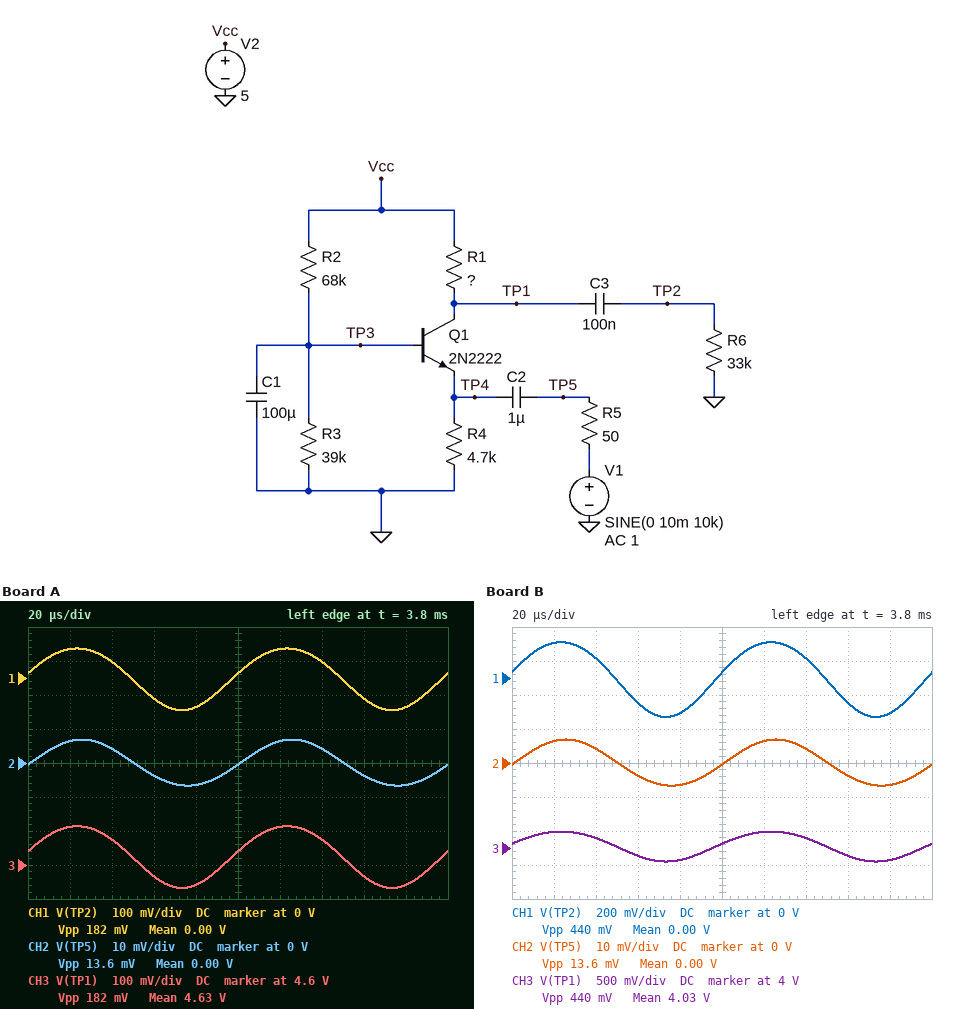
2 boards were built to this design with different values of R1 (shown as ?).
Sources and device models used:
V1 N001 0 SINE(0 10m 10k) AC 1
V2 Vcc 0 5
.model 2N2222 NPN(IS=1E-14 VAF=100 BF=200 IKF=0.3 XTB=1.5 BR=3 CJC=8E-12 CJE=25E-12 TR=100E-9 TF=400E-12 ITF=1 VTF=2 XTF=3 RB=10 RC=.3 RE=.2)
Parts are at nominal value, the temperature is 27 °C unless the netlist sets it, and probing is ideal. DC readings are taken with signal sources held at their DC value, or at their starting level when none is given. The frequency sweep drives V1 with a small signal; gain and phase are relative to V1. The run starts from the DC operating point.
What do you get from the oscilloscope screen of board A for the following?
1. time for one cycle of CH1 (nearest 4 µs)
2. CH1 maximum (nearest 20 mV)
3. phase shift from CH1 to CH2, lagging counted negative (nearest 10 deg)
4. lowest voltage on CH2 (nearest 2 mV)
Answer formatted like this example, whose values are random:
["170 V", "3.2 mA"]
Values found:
["100 µs", "80 mV", "-10 deg", "-6 mV"]
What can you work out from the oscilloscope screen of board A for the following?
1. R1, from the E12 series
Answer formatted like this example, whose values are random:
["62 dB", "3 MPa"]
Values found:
["1.5 kΩ"]
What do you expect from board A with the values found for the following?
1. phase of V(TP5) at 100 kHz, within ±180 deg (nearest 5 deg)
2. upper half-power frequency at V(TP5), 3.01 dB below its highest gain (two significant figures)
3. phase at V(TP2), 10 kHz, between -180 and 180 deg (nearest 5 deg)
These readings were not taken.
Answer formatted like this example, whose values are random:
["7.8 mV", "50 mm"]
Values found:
["0 deg", "3.3 kHz", "5 deg"]
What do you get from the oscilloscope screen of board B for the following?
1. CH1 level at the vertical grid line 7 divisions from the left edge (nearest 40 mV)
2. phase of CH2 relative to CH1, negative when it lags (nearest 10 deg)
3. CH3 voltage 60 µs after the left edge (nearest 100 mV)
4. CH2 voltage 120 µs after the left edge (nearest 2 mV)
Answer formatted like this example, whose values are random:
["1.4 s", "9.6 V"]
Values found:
["120 mV", "-10 deg", "3.9 V", "6 mV"]
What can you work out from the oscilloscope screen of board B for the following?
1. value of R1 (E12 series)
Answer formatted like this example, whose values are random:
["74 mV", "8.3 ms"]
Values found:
["3.9 kΩ"]
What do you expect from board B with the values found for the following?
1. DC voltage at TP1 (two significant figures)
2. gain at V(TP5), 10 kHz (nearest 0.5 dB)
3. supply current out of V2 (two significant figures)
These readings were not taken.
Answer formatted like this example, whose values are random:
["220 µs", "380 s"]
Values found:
["4.0 V", "-3.5 dB", "300 µA"]
